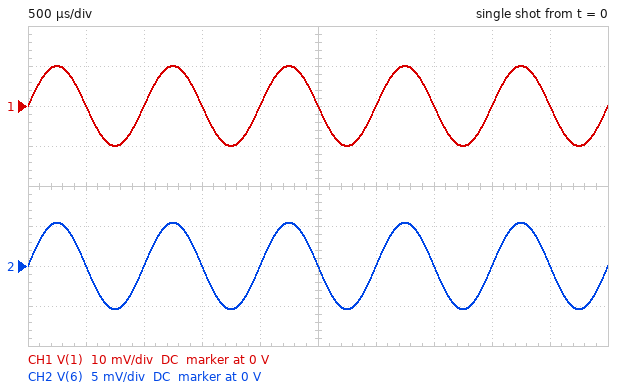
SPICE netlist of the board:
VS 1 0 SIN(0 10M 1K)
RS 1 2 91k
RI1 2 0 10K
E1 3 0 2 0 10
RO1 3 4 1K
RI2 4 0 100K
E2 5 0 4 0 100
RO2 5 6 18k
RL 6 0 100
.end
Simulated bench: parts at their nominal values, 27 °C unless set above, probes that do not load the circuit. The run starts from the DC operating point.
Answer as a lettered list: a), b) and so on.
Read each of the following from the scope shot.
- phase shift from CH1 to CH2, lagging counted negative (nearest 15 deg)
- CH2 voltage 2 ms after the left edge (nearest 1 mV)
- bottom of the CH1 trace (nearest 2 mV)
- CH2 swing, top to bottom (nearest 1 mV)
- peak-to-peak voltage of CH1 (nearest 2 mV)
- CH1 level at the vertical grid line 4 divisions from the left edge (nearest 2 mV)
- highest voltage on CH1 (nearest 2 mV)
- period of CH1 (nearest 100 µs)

a) 0 deg
b) 0 V
c) -10 mV
d) 11 mV
e) 20 mV
f) 0 V
g) 10 mV
h) 1.0 ms
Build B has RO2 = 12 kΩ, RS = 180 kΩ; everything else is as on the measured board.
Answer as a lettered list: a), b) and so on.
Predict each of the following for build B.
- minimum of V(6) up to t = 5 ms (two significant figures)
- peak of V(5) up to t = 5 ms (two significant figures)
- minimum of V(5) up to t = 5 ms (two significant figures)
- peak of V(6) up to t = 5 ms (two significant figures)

a) -4.3 mV
b) 520 mV
c) -520 mV
d) 4.3 mV
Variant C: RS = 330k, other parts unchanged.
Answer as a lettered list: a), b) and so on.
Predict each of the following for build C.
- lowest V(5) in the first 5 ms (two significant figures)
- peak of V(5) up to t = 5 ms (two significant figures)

a) -290 mV
b) 290 mV
